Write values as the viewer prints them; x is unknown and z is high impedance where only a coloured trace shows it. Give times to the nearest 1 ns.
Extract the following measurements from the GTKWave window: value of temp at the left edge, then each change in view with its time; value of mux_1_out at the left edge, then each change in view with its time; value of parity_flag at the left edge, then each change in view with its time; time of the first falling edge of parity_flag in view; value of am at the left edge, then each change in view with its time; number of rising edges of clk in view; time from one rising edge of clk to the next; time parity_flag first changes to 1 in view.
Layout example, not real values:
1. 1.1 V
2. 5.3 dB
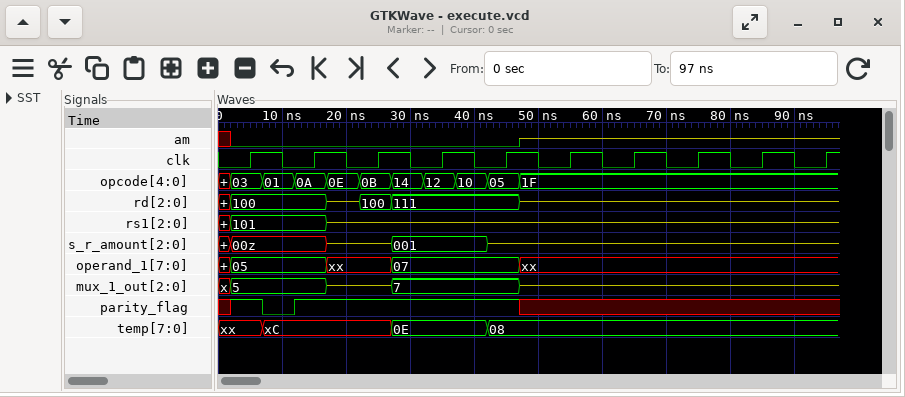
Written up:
1. xx, xC at 7 ns, 0E at 27 ns, 08 at 42 ns
2. x, 5 at 2 ns, z at 17 ns, 7 at 27 ns, z at 47 ns
3. x, 1 at 2 ns, 0 at 7 ns, 1 at 12 ns, x at 47 ns
4. 7 ns
5. x, 0 at 2 ns, z at 47 ns
6. 10
7. 10 ns
8. 2 ns
